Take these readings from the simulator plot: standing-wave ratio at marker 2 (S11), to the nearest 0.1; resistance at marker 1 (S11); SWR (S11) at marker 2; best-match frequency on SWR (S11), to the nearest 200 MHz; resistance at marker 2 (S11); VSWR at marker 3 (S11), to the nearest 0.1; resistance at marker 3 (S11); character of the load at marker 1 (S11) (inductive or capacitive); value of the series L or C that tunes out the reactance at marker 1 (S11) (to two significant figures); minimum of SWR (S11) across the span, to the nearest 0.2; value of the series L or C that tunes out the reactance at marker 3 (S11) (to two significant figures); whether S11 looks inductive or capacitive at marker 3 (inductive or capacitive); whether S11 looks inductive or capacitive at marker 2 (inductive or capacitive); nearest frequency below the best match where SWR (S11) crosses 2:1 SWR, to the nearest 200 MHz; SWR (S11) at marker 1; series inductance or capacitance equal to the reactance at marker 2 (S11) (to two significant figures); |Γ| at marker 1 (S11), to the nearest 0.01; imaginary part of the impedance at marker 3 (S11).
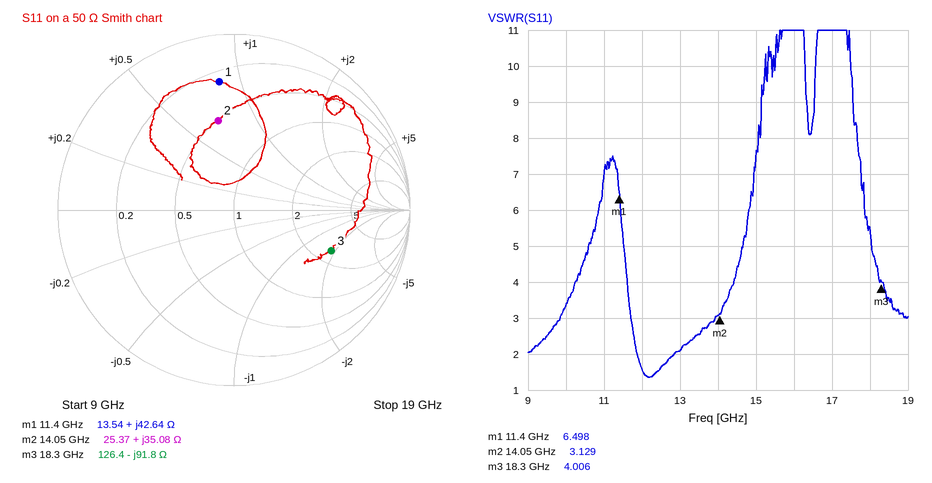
3.1
13.54 Ω
3.129
12.2 GHz
25.37 Ω
4.0
126.4 Ω
inductive
330 fF
1.4
800 pH
capacitive
inductive
11.8 GHz
6.498
400 pH
0.73
-91.8 Ω
